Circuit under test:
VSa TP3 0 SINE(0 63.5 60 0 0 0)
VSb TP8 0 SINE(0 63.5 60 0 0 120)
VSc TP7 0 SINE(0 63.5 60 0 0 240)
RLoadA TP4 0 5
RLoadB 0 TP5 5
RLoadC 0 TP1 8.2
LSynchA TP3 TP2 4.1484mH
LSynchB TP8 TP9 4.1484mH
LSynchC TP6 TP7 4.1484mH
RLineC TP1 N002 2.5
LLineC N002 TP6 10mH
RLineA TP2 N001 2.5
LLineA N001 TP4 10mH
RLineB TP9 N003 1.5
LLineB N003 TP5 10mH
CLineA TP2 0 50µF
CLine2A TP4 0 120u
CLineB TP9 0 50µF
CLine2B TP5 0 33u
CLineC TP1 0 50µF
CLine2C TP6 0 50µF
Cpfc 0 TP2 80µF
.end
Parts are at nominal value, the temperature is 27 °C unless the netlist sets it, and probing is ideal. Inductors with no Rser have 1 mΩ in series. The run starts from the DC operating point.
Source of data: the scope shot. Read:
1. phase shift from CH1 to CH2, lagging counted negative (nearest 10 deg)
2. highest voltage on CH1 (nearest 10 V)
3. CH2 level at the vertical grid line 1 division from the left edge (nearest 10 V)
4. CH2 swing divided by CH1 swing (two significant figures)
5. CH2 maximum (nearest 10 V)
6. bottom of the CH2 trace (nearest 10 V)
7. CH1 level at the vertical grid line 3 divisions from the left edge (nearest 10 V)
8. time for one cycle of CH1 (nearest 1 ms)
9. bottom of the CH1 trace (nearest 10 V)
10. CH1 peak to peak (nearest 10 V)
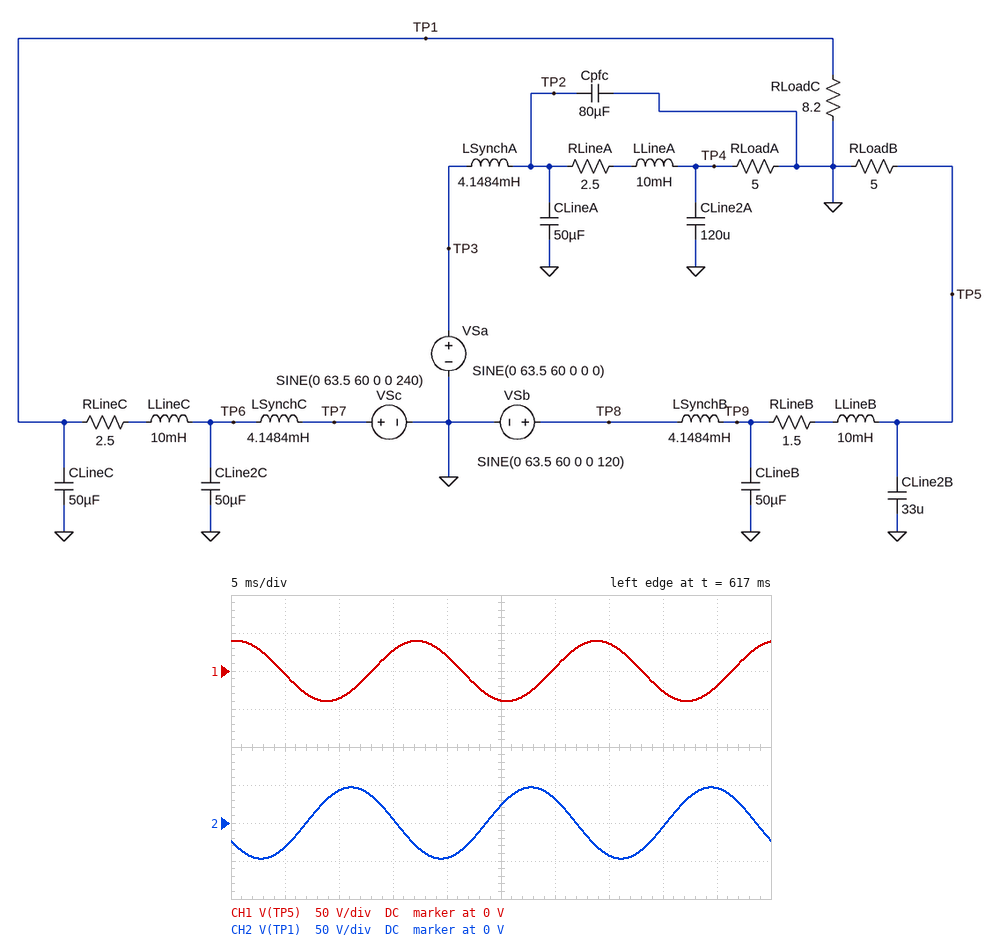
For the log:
130 deg
40 V
-30 V
1.2
50 V
-50 V
30 V
17 ms
-40 V
80 V
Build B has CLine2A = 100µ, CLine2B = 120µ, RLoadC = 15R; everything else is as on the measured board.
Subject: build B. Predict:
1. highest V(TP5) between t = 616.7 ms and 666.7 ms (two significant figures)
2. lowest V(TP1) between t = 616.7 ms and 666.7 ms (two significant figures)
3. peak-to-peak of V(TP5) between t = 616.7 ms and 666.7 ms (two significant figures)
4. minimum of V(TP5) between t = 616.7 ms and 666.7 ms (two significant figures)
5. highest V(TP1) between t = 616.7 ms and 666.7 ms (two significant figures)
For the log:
42 V
-57 V
84 V
-42 V
57 V
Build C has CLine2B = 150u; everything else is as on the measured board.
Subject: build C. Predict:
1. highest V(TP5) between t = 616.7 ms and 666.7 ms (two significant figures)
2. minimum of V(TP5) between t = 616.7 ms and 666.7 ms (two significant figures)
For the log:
43 V
-43 V
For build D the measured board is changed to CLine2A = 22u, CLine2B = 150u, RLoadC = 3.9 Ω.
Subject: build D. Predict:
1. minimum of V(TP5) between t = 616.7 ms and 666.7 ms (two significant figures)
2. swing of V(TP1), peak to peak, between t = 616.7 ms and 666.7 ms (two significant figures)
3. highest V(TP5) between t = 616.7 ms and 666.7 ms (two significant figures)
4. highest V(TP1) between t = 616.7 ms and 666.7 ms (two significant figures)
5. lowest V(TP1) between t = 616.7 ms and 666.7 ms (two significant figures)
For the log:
-43 V
62 V
43 V
31 V
-31 V
